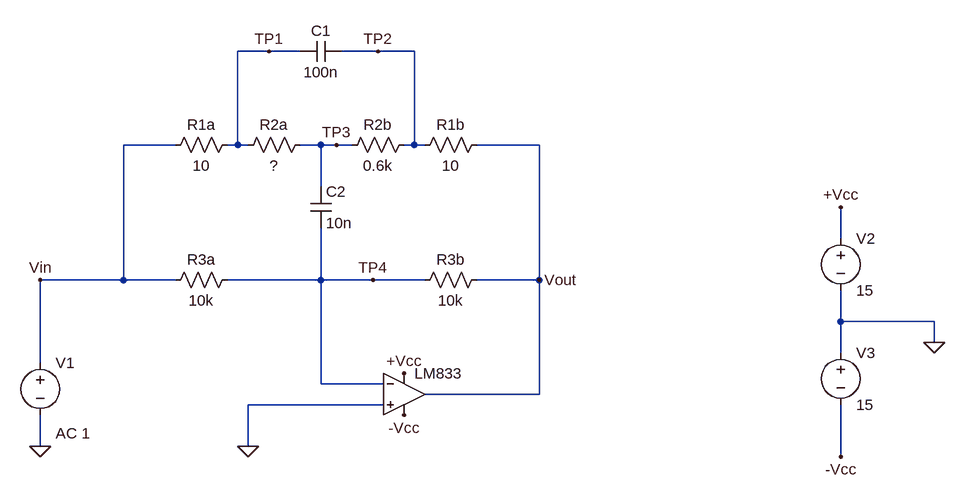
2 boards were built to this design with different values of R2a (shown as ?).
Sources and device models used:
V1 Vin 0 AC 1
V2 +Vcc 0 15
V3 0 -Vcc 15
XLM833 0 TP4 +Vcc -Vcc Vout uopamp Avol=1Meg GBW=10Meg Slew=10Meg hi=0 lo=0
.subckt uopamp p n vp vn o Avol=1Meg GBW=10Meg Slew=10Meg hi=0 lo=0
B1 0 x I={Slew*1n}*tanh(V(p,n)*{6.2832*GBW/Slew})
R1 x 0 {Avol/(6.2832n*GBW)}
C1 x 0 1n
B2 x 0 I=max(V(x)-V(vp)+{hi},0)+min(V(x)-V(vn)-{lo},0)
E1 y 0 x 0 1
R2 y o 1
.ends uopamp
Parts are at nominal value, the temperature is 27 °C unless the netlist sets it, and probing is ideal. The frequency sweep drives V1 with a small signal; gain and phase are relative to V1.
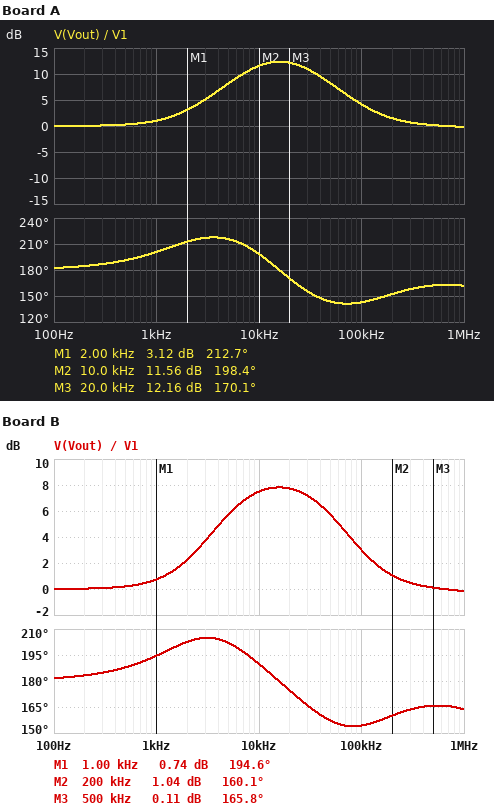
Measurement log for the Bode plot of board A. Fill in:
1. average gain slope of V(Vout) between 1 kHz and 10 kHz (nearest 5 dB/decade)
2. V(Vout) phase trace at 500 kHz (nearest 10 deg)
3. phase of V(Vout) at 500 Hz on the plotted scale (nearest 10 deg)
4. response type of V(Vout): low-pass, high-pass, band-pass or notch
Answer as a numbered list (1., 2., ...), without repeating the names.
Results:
1. 10 dB/decade
2. 160 deg
3. 190 deg
4. band-pass
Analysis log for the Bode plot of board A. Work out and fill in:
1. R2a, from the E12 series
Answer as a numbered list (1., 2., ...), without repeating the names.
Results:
1. 120 Ω
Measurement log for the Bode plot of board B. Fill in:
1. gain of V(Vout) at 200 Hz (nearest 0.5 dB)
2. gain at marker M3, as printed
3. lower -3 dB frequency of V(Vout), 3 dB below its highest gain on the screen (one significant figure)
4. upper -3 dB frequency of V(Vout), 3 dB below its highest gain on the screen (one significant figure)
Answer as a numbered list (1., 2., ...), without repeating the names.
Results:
1. 0 dB
2. 0.11 dB
3. 4 kHz
4. 60 kHz
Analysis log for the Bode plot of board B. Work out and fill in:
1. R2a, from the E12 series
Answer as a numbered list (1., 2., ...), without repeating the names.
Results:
1. 220 Ω
